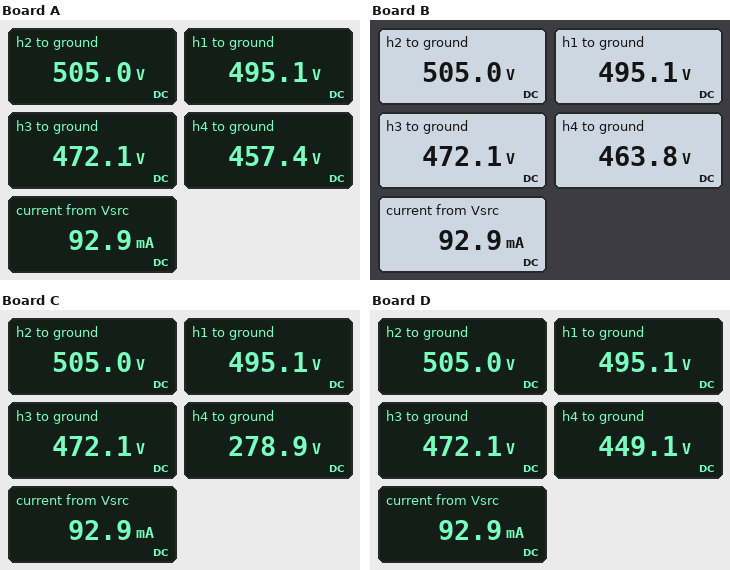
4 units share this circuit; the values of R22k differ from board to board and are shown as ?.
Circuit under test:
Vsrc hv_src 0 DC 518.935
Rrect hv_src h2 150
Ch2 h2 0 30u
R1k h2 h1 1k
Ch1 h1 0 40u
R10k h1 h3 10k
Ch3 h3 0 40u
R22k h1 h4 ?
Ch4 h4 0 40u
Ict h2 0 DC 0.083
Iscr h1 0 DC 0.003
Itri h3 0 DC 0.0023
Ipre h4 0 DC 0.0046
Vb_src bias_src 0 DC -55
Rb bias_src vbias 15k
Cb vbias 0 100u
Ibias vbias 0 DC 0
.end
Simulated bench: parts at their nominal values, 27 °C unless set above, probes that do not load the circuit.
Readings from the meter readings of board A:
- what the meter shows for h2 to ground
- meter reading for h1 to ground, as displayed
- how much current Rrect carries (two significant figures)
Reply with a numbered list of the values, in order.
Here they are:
1. 505.0 V
2. 495.1 V
3. 93 mA
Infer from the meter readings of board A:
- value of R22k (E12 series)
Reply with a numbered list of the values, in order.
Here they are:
1. 8.2 kΩ
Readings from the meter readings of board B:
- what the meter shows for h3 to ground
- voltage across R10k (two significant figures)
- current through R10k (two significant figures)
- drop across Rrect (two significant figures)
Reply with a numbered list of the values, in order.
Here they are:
1. 472.1 V
2. 23 V
3. 2.3 mA
4. 14 V
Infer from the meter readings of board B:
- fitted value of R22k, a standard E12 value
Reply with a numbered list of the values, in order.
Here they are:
1. 6.8 kΩ
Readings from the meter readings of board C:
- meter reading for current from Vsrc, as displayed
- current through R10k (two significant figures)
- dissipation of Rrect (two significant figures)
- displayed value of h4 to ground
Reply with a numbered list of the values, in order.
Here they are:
1. 92.9 mA
2. 2.3 mA
3. 1.3 W
4. 278.9 V
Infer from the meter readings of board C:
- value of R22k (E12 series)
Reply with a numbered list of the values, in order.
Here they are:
1. 47 kΩ
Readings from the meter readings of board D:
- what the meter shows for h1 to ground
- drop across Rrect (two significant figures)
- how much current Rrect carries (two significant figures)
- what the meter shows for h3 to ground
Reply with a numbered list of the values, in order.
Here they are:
1. 495.1 V
2. 14 V
3. 93 mA
4. 472.1 V
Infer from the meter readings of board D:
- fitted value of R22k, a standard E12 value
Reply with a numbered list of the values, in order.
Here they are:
1. 10 kΩ
